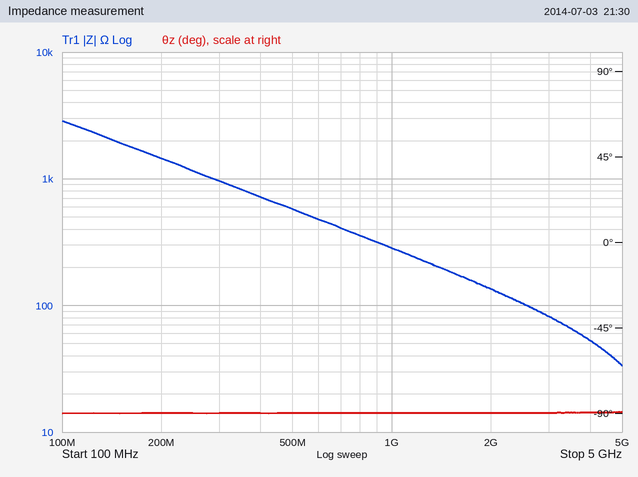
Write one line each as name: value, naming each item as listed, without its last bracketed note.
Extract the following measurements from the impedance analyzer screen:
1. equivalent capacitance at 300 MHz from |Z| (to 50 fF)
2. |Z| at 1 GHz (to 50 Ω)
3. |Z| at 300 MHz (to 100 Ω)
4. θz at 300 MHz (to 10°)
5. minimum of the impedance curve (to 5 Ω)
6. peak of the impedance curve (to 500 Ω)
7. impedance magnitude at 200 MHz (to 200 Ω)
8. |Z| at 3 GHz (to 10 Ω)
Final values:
equivalent capacitance at 300 MHz from |Z|: 550 fF
|Z| at 1 GHz: 300 Ω
|Z| at 300 MHz: 1.0 kΩ
θz at 300 MHz: -90°
minimum of the impedance curve: 35 Ω
peak of the impedance curve: 3.0 kΩ
impedance magnitude at 200 MHz: 1.4 kΩ
|Z| at 3 GHz: 80 Ω
